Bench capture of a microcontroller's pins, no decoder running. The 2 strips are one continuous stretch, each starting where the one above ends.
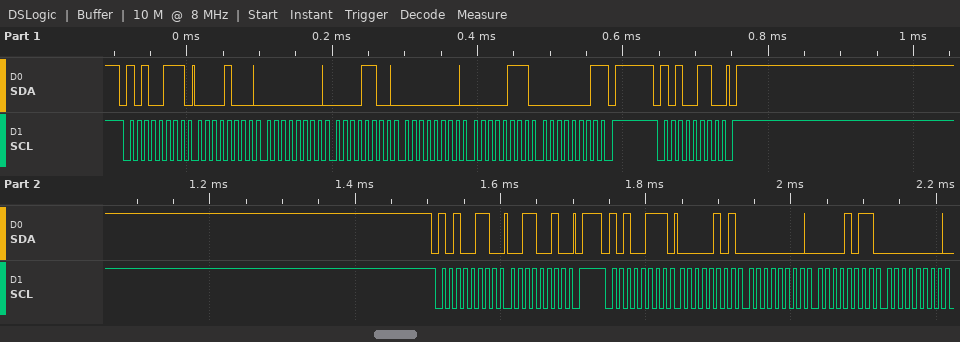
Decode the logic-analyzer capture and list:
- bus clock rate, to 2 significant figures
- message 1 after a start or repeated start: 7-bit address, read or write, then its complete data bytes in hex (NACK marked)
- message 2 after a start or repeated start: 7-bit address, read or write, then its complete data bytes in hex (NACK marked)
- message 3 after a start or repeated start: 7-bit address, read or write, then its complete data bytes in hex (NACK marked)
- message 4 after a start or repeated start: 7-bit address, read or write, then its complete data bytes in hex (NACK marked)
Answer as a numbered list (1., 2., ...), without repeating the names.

1. 100 kHz
2. 0x53 read: 08 00 0C 00 07 01 NACK
3. 0x53 write
4. 0x53 write: 32
5. 0x53 read: 05 00 0B 00
